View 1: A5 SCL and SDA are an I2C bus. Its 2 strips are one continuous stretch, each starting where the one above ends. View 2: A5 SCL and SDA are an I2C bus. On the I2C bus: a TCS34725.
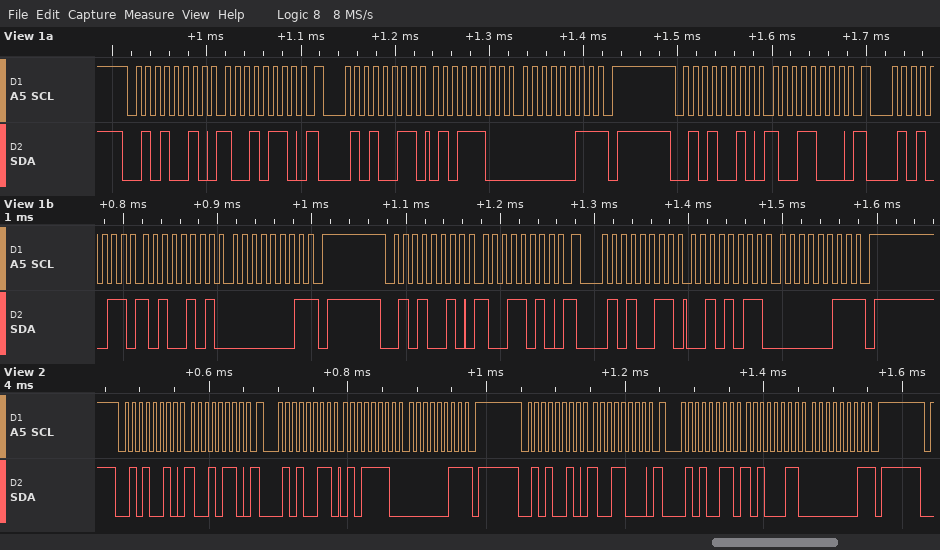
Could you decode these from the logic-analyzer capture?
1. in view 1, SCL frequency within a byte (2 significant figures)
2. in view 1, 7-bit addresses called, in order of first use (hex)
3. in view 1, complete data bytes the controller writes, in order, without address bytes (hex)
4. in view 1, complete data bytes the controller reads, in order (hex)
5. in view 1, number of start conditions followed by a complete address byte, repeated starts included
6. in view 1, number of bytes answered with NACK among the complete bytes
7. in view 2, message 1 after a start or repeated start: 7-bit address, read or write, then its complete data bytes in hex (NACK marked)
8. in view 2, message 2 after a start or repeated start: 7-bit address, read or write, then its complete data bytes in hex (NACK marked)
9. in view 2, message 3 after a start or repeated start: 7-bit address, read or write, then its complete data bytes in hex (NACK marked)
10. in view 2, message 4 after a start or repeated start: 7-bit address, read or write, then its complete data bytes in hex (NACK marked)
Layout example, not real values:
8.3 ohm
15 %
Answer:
100 kHz
0x29
96 98 9A
5C 03 A5 01 2B 03
6
3
0x29 write: 96
0x29 read: 5E 03 NACK
0x29 write: 98
0x29 read: A3 01 NACK
